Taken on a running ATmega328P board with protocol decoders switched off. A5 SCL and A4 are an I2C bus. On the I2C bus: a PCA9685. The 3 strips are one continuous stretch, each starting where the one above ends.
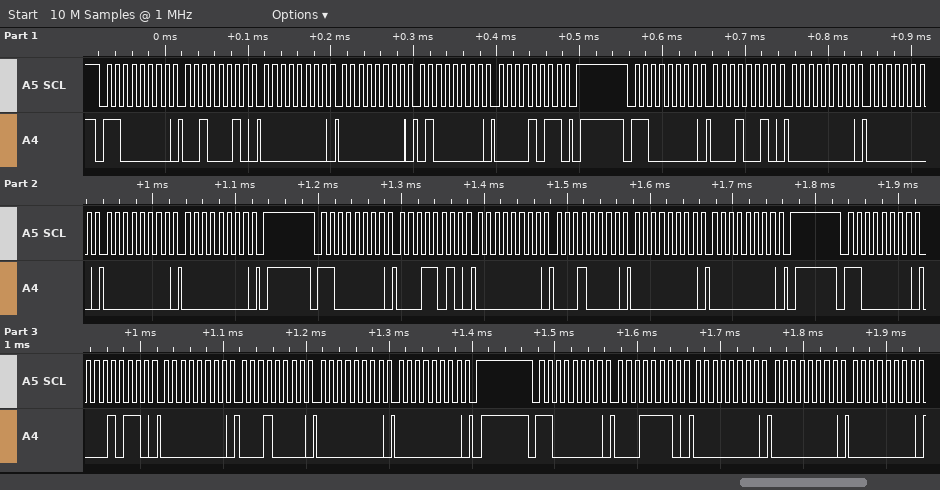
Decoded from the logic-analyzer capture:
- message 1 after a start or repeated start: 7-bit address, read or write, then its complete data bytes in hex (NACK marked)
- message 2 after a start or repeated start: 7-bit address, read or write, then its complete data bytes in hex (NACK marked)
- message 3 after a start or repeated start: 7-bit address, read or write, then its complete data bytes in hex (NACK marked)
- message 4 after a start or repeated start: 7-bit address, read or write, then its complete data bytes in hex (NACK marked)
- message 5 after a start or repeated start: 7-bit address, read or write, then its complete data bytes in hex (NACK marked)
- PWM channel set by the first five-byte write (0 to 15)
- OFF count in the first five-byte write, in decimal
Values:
0x60 write: 22 00 00 40 0B
0x60 write: 12 00 00 00 00
0x60 write: 1A 00 10 00 00
0x60 write: 16 00 10 00 00
0x60 write: 1E 00 00 00
7
2880
